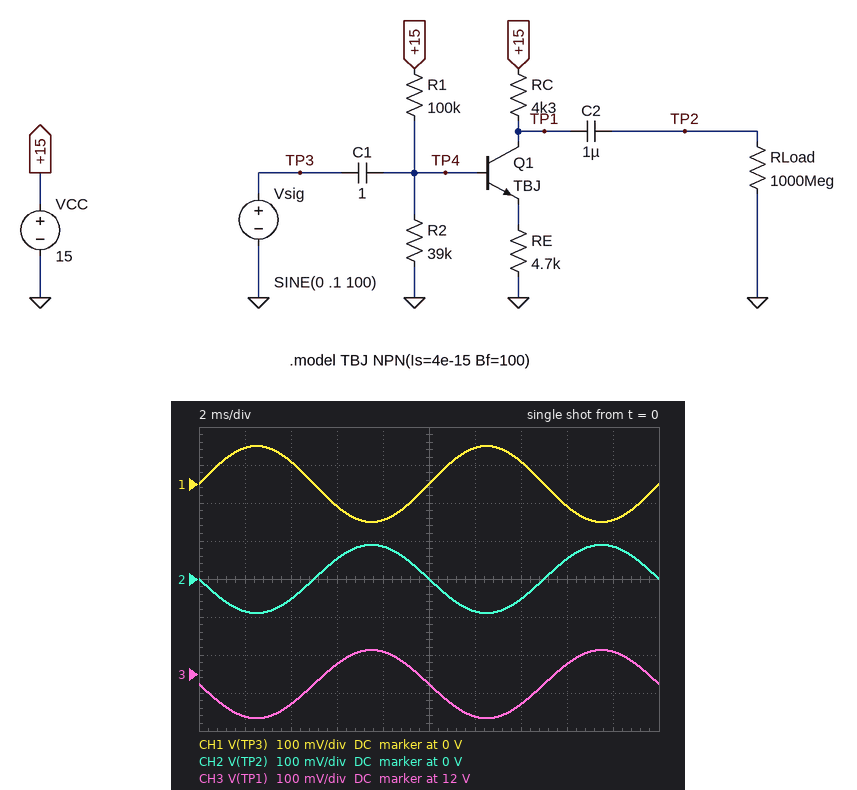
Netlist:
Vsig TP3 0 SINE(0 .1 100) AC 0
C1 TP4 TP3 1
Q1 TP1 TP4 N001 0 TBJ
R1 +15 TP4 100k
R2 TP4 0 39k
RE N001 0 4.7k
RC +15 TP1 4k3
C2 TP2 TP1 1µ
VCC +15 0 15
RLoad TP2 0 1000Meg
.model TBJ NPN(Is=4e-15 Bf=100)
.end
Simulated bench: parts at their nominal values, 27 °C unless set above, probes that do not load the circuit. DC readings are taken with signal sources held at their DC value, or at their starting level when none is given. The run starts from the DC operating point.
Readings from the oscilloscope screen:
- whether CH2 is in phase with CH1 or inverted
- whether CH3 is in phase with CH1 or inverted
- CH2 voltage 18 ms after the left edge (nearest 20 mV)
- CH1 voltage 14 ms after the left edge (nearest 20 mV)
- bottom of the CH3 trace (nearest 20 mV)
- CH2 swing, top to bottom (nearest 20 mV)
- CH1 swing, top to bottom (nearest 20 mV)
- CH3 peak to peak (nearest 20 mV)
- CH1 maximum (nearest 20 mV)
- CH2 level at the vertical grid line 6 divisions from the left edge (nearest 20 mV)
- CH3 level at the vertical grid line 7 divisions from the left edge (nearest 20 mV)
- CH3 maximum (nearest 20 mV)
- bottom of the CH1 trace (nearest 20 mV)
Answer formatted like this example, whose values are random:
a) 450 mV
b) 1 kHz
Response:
a) inverted
b) inverted
c) 80 mV
d) 60 mV
e) 11.88 V
f) 180 mV
g) 200 mV
h) 180 mV
i) 100 mV
j) -80 mV
k) 11.92 V
l) 12.06 V
m) -100 mV
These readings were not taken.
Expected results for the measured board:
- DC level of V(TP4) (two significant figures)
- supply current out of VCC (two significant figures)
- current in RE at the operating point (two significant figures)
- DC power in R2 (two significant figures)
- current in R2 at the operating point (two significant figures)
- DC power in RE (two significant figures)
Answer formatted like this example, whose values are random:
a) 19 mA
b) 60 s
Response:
a) 4.0 V
b) 810 µA
c) 710 µA
d) 410 µW
e) 100 µA
f) 2.4 mW
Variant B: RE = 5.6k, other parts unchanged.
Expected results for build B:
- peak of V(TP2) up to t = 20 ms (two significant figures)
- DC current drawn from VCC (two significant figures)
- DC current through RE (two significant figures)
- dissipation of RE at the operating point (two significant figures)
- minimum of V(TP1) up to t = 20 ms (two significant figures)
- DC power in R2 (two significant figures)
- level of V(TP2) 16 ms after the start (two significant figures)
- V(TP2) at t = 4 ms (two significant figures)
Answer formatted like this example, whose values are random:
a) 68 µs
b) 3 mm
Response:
a) 75 mV
b) 710 µA
c) 600 µA
d) 2.0 mW
e) 12 V
f) 420 µW
g) 44 mV
h) -44 mV
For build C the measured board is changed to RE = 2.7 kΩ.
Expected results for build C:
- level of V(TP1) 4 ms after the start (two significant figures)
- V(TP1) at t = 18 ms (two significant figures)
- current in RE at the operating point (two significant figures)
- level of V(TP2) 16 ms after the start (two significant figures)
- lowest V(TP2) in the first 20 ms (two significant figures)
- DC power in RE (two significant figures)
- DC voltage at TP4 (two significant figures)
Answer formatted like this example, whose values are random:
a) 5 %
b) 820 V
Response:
a) 9.9 V
b) 10 V
c) 1.2 mA
d) 92 mV
e) -160 mV
f) 3.8 mW
g) 3.9 V
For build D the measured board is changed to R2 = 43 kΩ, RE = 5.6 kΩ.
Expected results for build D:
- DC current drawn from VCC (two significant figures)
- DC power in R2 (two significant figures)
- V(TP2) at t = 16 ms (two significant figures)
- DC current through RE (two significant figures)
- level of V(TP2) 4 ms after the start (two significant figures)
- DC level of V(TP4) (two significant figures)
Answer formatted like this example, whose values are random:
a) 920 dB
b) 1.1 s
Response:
a) 750 µA
b) 430 µW
c) 44 mV
d) 650 µA
e) -44 mV
f) 4.3 V
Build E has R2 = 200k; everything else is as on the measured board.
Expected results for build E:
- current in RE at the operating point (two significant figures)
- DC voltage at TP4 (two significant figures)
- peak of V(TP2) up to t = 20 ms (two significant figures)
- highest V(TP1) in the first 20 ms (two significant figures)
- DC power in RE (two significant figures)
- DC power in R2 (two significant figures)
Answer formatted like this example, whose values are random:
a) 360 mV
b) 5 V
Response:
a) 1.7 mA
b) 8.5 V
c) 64 mV
d) 8.0 V
e) 13 mW
f) 360 µW
